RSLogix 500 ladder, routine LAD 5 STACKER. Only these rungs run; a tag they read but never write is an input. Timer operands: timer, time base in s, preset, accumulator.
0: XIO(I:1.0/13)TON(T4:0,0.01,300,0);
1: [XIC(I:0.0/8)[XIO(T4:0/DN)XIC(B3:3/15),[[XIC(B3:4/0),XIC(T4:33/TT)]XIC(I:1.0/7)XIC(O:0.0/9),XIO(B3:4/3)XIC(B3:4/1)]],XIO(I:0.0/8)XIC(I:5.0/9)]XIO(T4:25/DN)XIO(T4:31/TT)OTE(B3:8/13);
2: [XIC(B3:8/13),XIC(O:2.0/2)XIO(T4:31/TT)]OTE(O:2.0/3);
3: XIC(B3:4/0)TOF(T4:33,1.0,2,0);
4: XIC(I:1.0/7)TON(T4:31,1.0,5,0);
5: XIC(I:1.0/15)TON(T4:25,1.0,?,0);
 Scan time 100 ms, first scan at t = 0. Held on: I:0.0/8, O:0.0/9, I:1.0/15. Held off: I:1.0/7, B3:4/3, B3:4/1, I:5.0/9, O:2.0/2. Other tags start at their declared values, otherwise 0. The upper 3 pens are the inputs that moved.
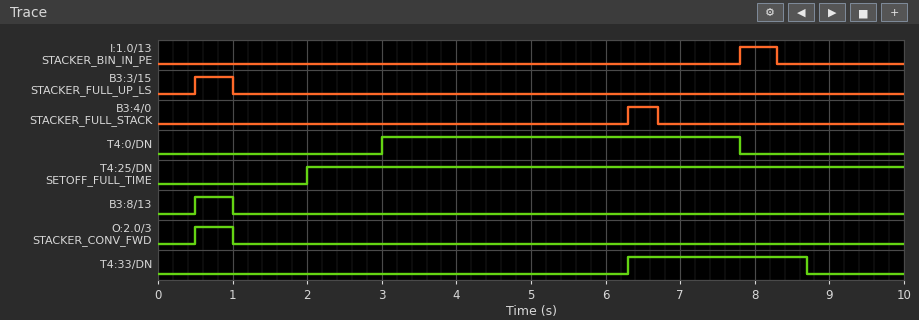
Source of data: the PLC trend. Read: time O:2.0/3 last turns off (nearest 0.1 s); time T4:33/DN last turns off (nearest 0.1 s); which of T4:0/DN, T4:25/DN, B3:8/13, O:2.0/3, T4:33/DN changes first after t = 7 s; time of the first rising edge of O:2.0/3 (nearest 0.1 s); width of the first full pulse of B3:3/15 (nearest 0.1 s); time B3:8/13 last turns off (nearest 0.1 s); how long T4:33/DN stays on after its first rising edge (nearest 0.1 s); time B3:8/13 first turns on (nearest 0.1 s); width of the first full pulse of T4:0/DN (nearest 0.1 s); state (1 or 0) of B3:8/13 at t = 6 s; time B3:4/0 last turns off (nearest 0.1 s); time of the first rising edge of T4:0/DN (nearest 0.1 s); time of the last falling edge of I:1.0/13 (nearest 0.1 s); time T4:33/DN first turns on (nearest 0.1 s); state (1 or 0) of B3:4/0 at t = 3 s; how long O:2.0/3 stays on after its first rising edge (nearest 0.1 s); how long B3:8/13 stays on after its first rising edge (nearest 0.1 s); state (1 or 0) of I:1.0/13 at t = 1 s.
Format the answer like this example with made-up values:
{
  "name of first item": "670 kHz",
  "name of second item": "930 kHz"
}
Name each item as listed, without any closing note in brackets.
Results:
{
  "time O:2.0/3 last turns off": "1.0 s",
  "time T4:33/DN last turns off": "8.7 s",
  "which of T4:0/DN, T4:25/DN, B3:8/13, O:2.0/3, T4:33/DN changes first after t = 7 s": "T4:0/DN",
  "time of the first rising edge of O:2.0/3": "0.5 s",
  "width of the first full pulse of B3:3/15": "0.5 s",
  "time B3:8/13 last turns off": "1.0 s",
  "how long T4:33/DN stays on after its first rising edge": "2.4 s",
  "time B3:8/13 first turns on": "0.5 s",
  "width of the first full pulse of T4:0/DN": "4.8 s",
  "state (1 or 0) of B3:8/13 at t = 6 s": "0",
  "time B3:4/0 last turns off": "6.7 s",
  "time of the first rising edge of T4:0/DN": "3.0 s",
  "time of the last falling edge of I:1.0/13": "8.3 s",
  "time T4:33/DN first turns on": "6.3 s",
  "state (1 or 0) of B3:4/0 at t = 3 s": "0",
  "how long O:2.0/3 stays on after its first rising edge": "0.5 s",
  "how long B3:8/13 stays on after its first rising edge": "0.5 s",
  "state (1 or 0) of I:1.0/13 at t = 1 s": "0"
}
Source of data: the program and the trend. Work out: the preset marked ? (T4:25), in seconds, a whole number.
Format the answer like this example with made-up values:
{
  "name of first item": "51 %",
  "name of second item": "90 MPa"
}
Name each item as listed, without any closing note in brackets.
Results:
{
  "the preset marked ? (T4:25), in seconds, a whole number": "2 s"
}
